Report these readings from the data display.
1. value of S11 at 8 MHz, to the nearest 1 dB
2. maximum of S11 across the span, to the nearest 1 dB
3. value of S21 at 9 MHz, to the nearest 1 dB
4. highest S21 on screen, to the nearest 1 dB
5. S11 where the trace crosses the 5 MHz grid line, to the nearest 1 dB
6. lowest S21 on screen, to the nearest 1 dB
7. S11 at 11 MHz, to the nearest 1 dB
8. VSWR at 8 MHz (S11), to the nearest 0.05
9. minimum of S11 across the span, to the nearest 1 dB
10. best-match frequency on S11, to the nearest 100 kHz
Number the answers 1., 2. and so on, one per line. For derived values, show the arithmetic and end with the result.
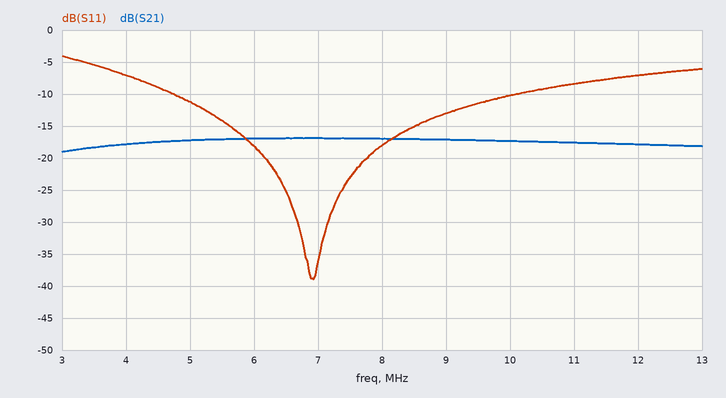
1. -18 dB
2. -4 dB
3. -17 dB
4. -17 dB
5. -11 dB
6. -19 dB
7. -8 dB
8. |Γ| = 10^(-18/20) = 0.1259; VSWR = (1 + 0.1259)/(1 − 0.1259) ≈ 1.29, so 1.30 to the nearest 0.05
9. -39 dB
10. 6.9 MHz
